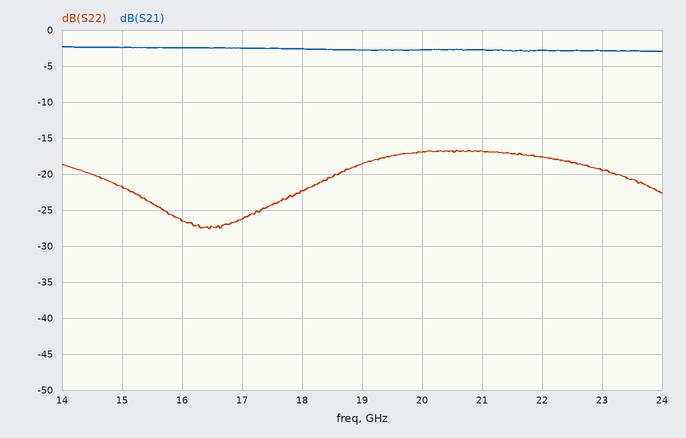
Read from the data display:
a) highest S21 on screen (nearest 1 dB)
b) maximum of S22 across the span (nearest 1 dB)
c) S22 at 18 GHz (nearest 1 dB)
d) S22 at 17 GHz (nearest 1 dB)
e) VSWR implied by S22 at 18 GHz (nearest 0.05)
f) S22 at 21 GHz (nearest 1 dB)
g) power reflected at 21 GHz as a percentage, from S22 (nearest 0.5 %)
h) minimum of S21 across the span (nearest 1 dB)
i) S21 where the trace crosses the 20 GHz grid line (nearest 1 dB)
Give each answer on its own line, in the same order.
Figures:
-2 dB
-17 dB
-22 dB
-26 dB
1.15
-17 dB
2.0 %
-3 dB
-3 dB
